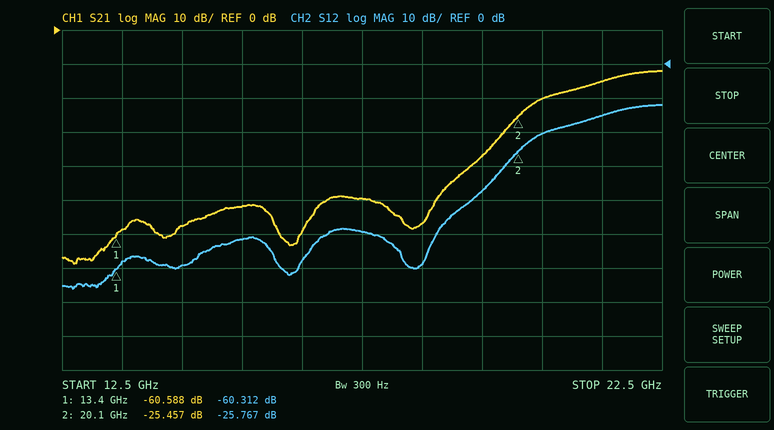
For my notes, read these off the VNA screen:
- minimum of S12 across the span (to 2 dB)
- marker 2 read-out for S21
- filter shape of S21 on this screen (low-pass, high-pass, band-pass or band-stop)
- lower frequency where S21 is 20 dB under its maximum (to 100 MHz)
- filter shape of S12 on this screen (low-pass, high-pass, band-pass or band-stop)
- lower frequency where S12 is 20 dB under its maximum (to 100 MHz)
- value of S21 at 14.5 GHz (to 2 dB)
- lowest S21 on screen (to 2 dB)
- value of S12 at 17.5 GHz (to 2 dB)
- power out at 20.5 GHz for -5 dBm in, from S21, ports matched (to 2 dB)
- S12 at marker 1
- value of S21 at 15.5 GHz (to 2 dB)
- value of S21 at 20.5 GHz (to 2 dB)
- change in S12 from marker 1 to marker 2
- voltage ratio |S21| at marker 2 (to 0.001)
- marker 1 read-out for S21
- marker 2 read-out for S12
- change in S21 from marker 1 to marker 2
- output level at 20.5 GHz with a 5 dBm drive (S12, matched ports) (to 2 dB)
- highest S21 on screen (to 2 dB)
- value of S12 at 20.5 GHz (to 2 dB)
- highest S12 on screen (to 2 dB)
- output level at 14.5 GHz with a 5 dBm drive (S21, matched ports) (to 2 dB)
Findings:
-66 dB
-25.457 dB
high-pass
19.8 GHz
high-pass
19.8 GHz
-58 dB
-68 dB
-50 dB
-26 dBm
-60.312 dB
-52 dB
-20 dB
34.545 dB
0.053
-60.588 dB
-25.767 dB
35.131 dB
-16 dBm
-12 dB
-20 dB
-12 dB
-52 dBm
